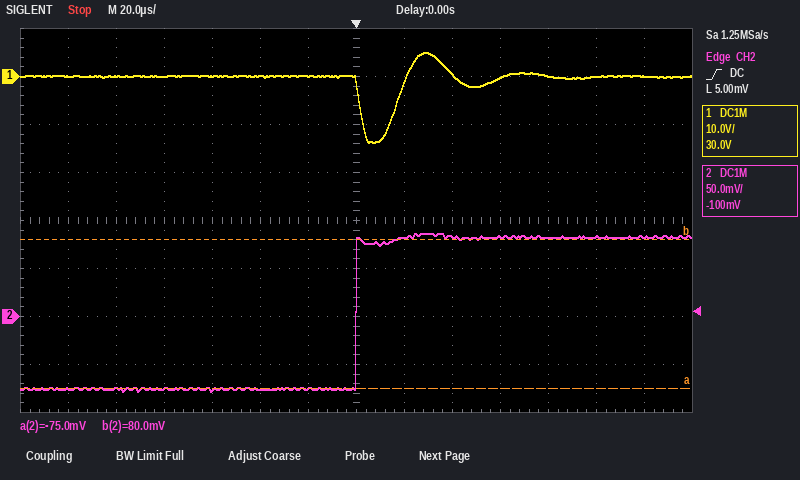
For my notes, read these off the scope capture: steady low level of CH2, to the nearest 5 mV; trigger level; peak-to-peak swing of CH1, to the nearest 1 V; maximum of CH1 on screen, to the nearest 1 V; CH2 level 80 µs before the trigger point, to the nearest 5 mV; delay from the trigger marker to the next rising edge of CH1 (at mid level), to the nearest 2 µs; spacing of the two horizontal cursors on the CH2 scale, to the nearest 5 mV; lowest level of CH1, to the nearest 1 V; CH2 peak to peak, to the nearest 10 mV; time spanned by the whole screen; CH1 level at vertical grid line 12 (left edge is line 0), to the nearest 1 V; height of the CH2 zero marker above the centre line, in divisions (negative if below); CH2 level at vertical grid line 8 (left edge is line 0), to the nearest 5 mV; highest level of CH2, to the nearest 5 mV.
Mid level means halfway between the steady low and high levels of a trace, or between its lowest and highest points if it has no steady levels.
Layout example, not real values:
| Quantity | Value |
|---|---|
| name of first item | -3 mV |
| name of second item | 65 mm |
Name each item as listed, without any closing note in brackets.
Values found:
| Quantity | Value |
|---|---|
| steady low level of CH2, to the nearest 5 mV | -75 mV |
| trigger level | 5.00 mV |
| peak-to-peak swing of CH1, to the nearest 1 V | 19 V |
| maximum of CH1 on screen, to the nearest 1 V | 5 V |
| CH2 level 80 µs before the trigger point, to the nearest 5 mV | -75 mV |
| delay from the trigger marker to the next rising edge of CH1 (at mid level), to the nearest 2 µs | 18 µs |
| spacing of the two horizontal cursors on the CH2 scale, to the nearest 5 mV | 155 mV |
| lowest level of CH1, to the nearest 1 V | -14 V |
| CH2 peak to peak, to the nearest 10 mV | 160 mV |
| time spanned by the whole screen | 280 µs |
| CH1 level at vertical grid line 12 (left edge is line 0), to the nearest 1 V | 0 V |
| height of the CH2 zero marker above the centre line, in divisions | -2.0 div |
| CH2 level at vertical grid line 8 (left edge is line 0), to the nearest 5 mV | 80 mV |
| highest level of CH2, to the nearest 5 mV | 85 mV |
